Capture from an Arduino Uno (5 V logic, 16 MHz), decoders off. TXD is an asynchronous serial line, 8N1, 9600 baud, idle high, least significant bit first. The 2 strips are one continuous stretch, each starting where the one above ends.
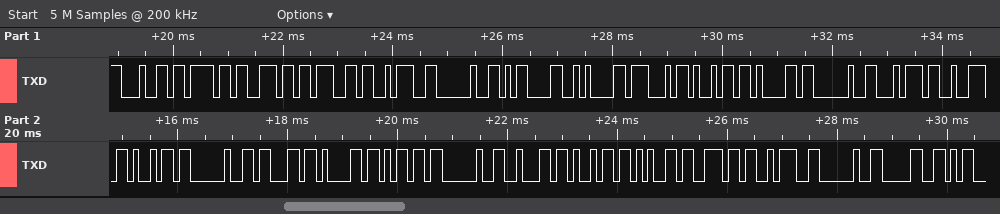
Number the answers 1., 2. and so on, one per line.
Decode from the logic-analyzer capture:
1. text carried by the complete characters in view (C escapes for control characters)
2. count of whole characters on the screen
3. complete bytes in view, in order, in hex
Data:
1. "dong: \r\nGia tri cam bien: 0"
2. 27
3. 0x64 0x6F 0x6E 0x67 0x3A 0x20 0x0D 0x0A 0x47 0x69 0x61 0x20 0x74 0x72 0x69 0x20 0x63 0x61 0x6D 0x20 0x62 0x69 0x65 0x6E 0x3A 0x20 0x30
